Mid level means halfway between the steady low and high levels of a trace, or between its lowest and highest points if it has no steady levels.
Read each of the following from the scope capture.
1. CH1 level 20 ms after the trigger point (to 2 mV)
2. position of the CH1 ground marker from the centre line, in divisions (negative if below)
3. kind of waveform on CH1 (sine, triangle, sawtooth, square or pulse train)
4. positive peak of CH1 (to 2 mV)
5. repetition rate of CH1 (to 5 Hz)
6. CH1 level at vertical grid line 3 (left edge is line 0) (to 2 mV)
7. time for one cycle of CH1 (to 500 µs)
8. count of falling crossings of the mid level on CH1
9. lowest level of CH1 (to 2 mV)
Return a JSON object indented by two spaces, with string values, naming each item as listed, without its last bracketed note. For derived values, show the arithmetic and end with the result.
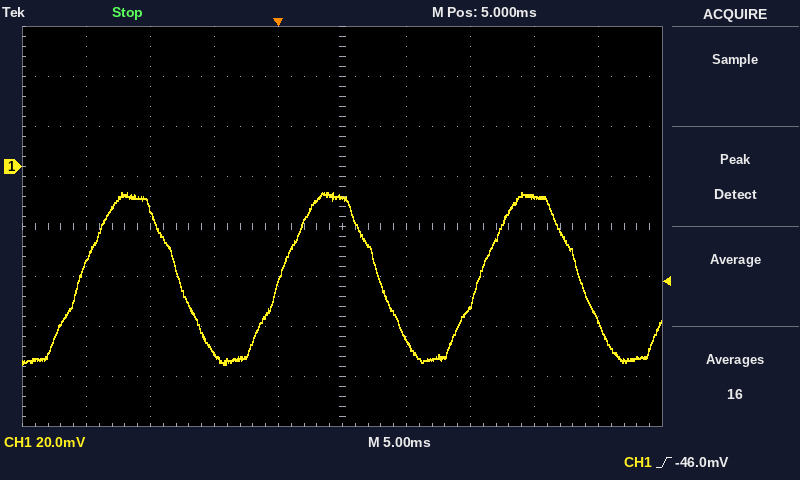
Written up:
{
  "CH1 level 20 ms after the trigger point": "-12 mV",
  "position of the CH1 ground marker from the centre line, in divisions": "+1.2 div",
  "kind of waveform on CH1": "sine",
  "positive peak of CH1": "-10 mV",
  "repetition rate of CH1": "1 / 15.5 ms ≈ 65 Hz",
  "CH1 level at vertical grid line 3 (left edge is line 0)": "-74 mV",
  "time for one cycle of CH1": "15.5 ms",
  "count of falling crossings of the mid level on CH1": "3",
  "lowest level of CH1": "-80 mV"
}
